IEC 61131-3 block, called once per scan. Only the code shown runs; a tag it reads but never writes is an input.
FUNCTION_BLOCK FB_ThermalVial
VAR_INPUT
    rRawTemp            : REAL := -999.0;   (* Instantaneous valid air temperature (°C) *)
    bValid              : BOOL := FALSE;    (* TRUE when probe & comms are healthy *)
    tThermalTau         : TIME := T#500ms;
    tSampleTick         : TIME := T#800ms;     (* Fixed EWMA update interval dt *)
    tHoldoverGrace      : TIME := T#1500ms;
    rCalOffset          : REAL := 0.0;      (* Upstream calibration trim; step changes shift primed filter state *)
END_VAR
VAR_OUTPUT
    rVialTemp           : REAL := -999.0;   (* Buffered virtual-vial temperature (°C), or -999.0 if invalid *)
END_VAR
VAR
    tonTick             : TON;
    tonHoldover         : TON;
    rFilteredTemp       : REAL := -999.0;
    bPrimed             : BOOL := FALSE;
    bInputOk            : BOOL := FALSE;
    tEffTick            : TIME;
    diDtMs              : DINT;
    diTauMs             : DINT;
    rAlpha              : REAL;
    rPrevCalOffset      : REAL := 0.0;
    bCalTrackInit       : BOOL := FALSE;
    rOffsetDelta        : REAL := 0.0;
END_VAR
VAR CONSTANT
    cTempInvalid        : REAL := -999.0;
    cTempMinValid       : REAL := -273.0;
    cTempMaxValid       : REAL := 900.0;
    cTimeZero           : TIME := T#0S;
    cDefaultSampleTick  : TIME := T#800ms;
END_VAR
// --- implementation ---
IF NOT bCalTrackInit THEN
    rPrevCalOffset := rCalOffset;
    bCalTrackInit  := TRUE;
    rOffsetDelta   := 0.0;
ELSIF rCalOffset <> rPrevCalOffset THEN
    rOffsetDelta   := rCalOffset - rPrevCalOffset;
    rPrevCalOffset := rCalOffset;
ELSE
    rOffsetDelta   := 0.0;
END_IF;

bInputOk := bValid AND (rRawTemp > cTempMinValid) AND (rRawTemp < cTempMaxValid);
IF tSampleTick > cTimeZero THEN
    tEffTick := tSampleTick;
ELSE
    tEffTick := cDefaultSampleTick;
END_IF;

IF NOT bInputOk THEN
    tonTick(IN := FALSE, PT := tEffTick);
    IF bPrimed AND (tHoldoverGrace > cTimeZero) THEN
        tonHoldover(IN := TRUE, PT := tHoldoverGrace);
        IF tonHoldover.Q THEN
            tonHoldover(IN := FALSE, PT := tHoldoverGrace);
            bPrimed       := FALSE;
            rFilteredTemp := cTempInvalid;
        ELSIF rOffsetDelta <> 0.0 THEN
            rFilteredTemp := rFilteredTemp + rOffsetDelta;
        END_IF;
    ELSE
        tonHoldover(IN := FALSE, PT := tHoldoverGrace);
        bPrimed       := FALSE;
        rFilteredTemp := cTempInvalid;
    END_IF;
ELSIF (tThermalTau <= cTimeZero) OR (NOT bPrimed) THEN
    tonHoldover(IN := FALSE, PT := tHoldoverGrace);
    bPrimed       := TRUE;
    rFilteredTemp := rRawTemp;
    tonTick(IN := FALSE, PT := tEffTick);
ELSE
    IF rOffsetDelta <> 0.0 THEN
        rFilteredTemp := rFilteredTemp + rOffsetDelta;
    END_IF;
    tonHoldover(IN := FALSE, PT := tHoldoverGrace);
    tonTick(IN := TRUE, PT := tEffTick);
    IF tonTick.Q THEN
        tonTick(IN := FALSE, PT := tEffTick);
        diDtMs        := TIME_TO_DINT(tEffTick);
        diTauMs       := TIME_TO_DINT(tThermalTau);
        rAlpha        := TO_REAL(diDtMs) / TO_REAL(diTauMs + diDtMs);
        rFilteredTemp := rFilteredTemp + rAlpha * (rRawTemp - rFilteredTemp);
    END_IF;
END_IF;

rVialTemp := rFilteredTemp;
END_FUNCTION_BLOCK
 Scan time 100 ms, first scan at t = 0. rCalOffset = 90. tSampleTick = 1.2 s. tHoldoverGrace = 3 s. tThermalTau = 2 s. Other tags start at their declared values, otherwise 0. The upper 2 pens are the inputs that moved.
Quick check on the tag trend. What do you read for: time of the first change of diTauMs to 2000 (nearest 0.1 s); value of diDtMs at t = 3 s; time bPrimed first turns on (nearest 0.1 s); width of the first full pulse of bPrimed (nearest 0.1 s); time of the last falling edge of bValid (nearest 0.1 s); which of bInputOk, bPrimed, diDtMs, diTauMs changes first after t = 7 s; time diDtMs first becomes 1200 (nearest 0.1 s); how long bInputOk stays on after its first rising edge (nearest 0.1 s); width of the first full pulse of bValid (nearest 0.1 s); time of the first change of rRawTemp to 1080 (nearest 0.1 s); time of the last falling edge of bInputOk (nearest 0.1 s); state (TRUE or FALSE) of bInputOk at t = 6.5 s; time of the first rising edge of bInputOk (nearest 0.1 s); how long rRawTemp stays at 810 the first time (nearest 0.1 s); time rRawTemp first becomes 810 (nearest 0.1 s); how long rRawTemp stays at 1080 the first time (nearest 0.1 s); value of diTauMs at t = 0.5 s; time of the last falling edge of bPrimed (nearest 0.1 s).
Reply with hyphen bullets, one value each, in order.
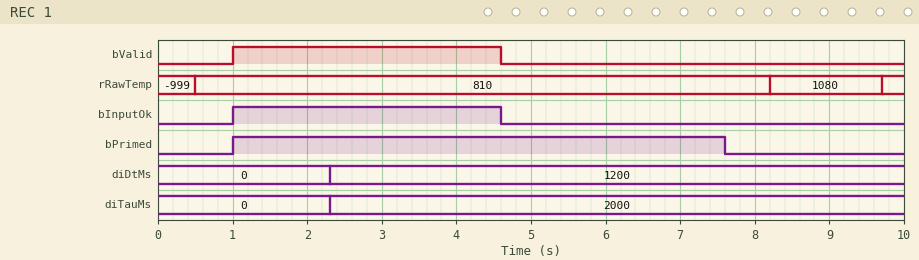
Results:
- 2.3 s
- 1200
- 1.0 s
- 6.6 s
- 4.6 s
- bPrimed
- 2.3 s
- 3.6 s
- 3.6 s
- 8.2 s
- 4.6 s
- FALSE
- 1.0 s
- 7.7 s
- 0.5 s
- 1.5 s
- 0
- 7.6 s
